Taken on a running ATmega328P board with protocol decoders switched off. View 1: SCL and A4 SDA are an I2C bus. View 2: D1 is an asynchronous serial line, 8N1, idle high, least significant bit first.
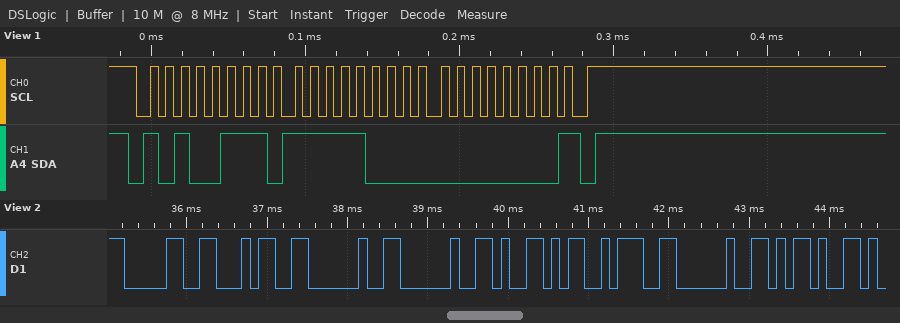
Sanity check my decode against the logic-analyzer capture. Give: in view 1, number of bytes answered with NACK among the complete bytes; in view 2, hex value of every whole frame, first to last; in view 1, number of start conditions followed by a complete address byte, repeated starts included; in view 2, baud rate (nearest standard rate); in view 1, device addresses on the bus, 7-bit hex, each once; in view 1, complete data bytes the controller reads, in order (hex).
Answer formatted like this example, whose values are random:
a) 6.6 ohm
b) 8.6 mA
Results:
a) 1
b) 0x30 0x34 0x20 0x20 0x59 0x3A 0x20 0x2D
c) 1
d) 9600 baud
e) 0x53
f) F8 00
